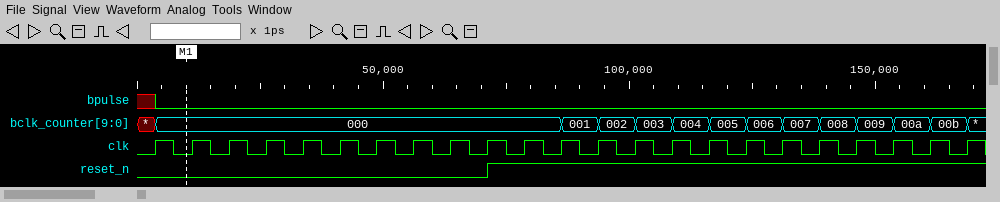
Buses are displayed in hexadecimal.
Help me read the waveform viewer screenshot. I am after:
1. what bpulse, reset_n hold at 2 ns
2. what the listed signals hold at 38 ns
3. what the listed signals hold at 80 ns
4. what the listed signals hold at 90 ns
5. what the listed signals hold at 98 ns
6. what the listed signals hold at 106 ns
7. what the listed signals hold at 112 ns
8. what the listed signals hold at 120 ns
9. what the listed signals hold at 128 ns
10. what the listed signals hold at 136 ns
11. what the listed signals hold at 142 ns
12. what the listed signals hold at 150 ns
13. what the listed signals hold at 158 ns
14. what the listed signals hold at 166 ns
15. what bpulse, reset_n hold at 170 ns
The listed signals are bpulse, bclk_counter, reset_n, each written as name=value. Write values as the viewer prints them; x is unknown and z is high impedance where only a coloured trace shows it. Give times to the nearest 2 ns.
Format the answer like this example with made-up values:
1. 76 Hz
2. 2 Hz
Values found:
1. bpulse=x, reset_n=0
2. bpulse=0, bclk_counter=000, reset_n=0
3. bpulse=0, bclk_counter=000, reset_n=1
4. bpulse=0, bclk_counter=001, reset_n=1
5. bpulse=0, bclk_counter=002, reset_n=1
6. bpulse=0, bclk_counter=003, reset_n=1
7. bpulse=0, bclk_counter=004, reset_n=1
8. bpulse=0, bclk_counter=005, reset_n=1
9. bpulse=0, bclk_counter=006, reset_n=1
10. bpulse=0, bclk_counter=007, reset_n=1
11. bpulse=0, bclk_counter=008, reset_n=1
12. bpulse=0, bclk_counter=009, reset_n=1
13. bpulse=0, bclk_counter=00a, reset_n=1
14. bpulse=0, bclk_counter=00b, reset_n=1
15. bpulse=0, reset_n=1
